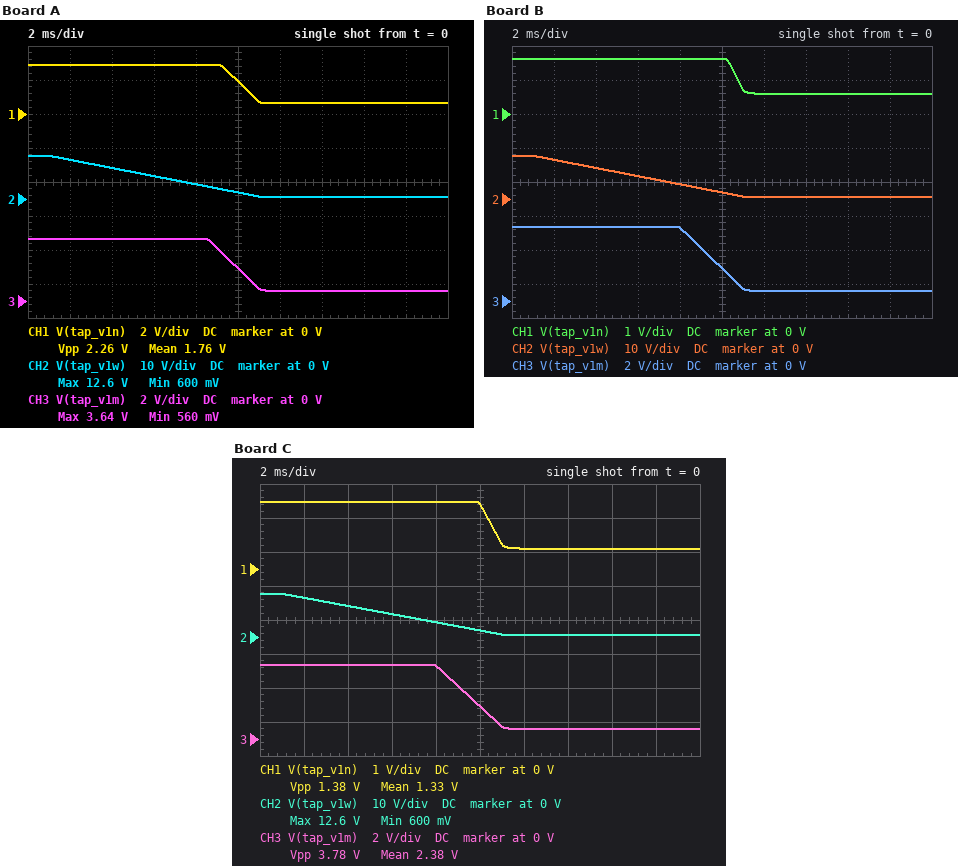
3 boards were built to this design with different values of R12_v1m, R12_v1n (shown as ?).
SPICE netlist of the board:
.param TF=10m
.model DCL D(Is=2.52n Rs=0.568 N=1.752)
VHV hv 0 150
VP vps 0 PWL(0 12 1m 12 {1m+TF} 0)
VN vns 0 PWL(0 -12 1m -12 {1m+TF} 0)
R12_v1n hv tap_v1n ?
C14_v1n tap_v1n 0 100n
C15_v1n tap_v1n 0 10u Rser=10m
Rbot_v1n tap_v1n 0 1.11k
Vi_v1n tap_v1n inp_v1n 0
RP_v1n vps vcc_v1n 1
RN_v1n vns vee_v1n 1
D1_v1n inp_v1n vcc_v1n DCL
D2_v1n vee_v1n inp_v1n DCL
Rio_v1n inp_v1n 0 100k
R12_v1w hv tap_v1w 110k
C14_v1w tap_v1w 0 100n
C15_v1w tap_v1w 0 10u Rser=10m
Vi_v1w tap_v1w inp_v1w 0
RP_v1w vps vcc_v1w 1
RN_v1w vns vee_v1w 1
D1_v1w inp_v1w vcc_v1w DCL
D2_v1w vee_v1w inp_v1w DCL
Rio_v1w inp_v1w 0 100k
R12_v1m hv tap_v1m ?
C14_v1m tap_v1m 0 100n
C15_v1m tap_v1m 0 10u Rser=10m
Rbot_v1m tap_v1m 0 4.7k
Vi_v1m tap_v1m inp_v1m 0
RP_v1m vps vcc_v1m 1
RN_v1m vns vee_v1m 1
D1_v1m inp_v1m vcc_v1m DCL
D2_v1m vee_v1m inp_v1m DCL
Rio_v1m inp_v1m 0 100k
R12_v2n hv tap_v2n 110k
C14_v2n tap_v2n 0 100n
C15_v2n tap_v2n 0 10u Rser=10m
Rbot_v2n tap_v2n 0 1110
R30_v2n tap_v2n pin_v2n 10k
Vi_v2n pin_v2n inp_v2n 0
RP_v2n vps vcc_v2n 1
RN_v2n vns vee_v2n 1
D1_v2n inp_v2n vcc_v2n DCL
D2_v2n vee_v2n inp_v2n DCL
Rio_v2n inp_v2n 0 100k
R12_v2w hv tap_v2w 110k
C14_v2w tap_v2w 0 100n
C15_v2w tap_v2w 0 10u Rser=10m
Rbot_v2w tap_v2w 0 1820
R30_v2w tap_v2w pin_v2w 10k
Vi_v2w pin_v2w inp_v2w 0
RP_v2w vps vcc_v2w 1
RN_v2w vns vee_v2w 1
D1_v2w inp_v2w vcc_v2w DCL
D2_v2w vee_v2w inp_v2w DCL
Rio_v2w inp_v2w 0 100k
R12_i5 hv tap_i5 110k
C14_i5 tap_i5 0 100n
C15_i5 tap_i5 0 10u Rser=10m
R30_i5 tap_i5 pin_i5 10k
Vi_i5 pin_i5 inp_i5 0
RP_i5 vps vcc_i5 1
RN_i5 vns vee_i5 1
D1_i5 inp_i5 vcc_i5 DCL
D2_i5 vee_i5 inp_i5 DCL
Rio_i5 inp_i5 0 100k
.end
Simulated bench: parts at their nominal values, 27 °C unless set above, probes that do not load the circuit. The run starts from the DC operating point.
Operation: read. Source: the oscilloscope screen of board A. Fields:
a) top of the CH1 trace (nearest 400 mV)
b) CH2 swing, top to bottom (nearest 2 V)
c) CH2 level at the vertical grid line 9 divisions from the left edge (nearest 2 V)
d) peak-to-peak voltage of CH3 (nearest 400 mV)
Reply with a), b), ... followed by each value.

a) 2.8 V
b) 12 V
c) 0 V
d) 3.2 V
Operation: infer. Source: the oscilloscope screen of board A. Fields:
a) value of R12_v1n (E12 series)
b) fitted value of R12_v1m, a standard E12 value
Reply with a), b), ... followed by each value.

a) 56 kΩ
b) 180 kΩ
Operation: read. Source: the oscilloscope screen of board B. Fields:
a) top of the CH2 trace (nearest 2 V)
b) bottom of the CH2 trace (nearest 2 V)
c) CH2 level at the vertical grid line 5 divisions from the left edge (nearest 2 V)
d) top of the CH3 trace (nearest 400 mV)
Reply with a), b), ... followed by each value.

a) 12 V
b) 0 V
c) 2 V
d) 4.4 V
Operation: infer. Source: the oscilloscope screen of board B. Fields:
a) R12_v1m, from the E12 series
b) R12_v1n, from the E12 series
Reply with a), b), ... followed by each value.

a) 150 kΩ
b) 100 kΩ
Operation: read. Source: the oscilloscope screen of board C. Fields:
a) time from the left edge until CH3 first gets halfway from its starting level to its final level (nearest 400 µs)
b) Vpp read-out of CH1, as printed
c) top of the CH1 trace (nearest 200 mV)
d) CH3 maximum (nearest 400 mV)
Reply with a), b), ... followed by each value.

a) 9.6 ms
b) 1.38 V
c) 2.0 V
d) 4.4 V
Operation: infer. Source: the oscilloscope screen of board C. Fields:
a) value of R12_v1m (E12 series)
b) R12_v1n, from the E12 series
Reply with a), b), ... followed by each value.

a) 150 kΩ
b) 82 kΩ
